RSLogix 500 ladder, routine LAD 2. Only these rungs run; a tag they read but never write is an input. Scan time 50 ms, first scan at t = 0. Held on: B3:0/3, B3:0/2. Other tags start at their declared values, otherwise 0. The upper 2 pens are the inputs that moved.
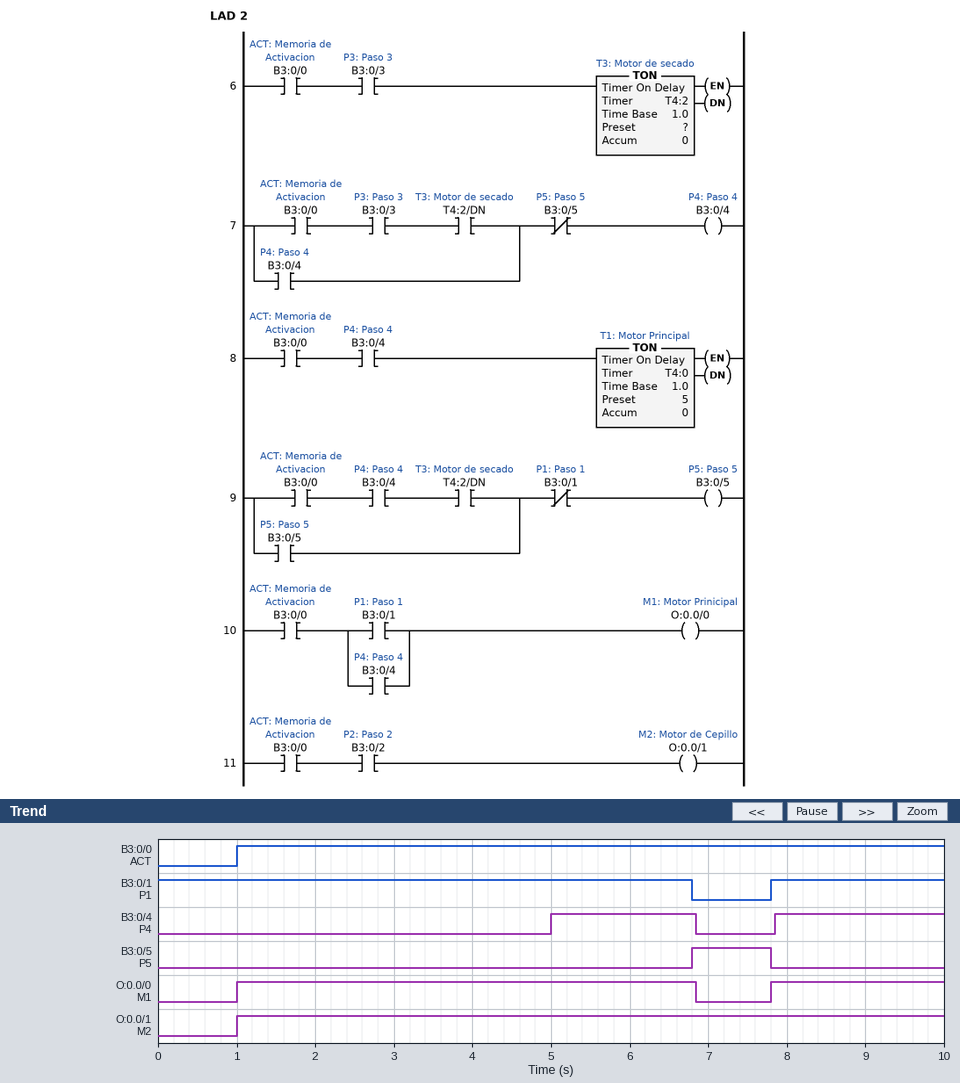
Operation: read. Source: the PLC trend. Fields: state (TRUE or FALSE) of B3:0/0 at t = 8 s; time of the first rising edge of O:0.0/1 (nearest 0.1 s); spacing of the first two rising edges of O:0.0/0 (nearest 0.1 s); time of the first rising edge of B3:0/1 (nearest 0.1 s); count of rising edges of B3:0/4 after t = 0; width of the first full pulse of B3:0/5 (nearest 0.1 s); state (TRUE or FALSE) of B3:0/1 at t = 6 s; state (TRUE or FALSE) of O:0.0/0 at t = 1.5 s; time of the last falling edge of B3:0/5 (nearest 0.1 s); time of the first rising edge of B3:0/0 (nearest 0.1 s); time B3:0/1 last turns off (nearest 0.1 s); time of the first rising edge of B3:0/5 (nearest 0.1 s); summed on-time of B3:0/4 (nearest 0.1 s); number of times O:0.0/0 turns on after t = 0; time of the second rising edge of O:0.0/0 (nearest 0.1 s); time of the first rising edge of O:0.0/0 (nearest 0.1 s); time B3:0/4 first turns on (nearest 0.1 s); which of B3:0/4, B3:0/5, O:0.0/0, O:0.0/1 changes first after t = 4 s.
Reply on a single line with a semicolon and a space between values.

TRUE; 1.0 s; 6.8 s; 7.8 s; 2; 1.0 s; TRUE; TRUE; 7.8 s; 1.0 s; 6.8 s; 6.8 s; 4.0 s; 2; 7.8 s; 1.0 s; 5.0 s; B3:0/4
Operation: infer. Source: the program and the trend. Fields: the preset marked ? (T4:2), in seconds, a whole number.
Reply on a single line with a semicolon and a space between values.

4 s
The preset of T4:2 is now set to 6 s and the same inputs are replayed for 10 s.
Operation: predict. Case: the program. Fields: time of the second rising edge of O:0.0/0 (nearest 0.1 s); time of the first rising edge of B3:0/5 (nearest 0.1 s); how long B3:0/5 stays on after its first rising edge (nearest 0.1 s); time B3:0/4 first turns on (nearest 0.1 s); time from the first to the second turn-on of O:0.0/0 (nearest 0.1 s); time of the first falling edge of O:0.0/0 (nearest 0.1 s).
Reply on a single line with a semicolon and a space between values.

7.0 s; 7.0 s; 0.8 s; 7.0 s; 6.0 s; 6.8 s
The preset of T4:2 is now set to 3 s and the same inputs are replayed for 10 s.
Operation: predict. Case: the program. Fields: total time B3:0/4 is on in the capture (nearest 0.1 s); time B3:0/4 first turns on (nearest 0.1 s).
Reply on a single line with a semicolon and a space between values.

5.0 s; 4.0 s
